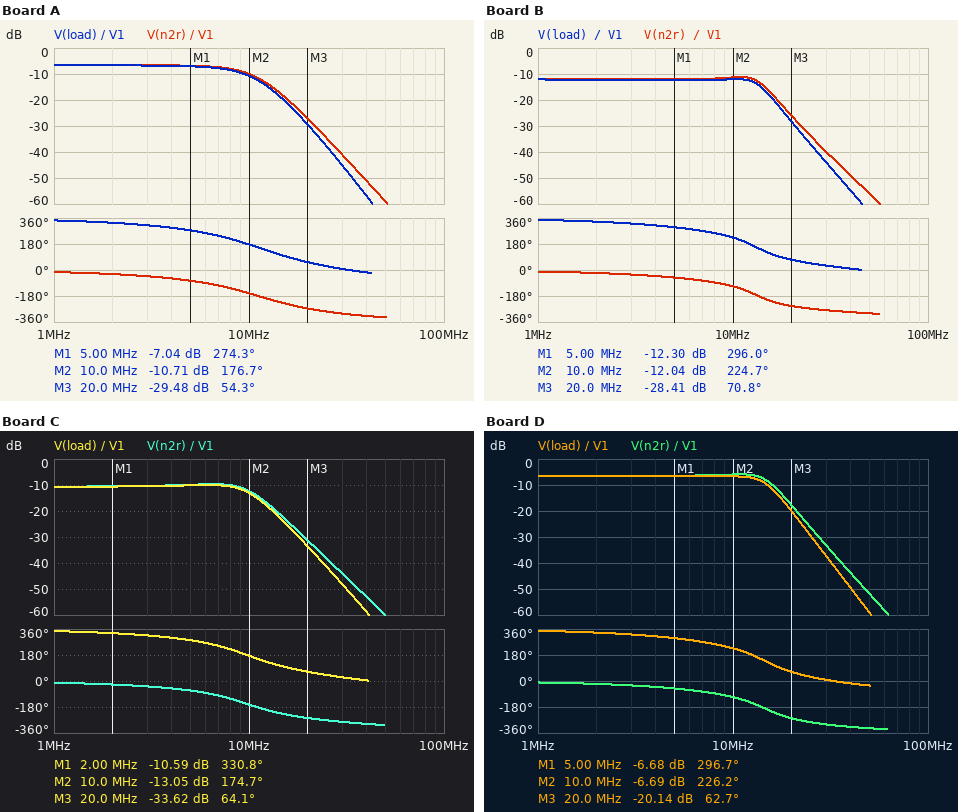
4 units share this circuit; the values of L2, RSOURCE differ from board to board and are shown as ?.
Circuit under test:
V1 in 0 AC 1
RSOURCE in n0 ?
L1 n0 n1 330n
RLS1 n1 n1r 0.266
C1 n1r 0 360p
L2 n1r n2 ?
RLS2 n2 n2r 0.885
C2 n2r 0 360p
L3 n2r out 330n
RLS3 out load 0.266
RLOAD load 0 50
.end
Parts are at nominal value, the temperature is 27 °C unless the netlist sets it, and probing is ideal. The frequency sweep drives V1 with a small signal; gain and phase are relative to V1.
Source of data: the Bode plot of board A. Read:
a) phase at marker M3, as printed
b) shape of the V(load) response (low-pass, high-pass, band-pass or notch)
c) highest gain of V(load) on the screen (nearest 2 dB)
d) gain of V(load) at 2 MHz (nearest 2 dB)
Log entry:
54.3 deg
low-pass
-6 dB
-6 dB
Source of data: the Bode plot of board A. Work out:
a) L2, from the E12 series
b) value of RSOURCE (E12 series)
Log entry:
2.2 µH
56 Ω
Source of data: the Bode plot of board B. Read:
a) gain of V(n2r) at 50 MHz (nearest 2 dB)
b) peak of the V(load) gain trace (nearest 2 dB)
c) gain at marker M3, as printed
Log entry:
-56 dB
-12 dB
-28.41 dB
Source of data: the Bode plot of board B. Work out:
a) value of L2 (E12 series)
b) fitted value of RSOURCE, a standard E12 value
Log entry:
1 µH
150 Ω
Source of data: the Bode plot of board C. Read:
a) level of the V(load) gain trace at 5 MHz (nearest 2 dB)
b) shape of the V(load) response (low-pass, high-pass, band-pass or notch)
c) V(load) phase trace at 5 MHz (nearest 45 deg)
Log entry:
-10 dB
low-pass
270 deg
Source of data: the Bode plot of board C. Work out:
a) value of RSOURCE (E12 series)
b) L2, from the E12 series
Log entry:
120 Ω
1.8 µH
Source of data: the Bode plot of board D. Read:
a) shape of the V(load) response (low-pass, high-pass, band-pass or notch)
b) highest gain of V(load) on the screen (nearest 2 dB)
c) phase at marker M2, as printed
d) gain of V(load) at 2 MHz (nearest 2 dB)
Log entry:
low-pass
-6 dB
226.2 deg
-6 dB
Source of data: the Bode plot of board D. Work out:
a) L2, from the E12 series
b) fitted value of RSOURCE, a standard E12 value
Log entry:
1 µH
56 Ω
